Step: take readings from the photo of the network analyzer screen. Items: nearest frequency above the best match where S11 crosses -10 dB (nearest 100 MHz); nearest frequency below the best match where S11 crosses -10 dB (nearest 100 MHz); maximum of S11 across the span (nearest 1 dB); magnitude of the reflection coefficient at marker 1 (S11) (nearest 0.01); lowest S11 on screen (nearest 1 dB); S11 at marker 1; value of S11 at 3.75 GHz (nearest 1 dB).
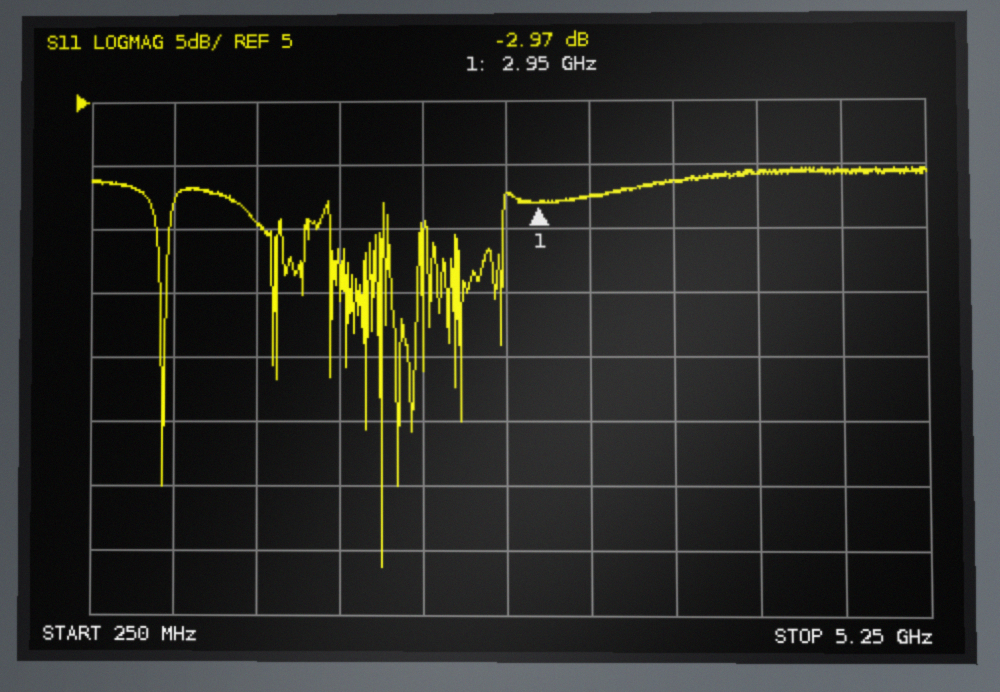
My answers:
2.0 GHz
2.0 GHz
0 dB
0.71
-31 dB
-2.97 dB
-1 dB
